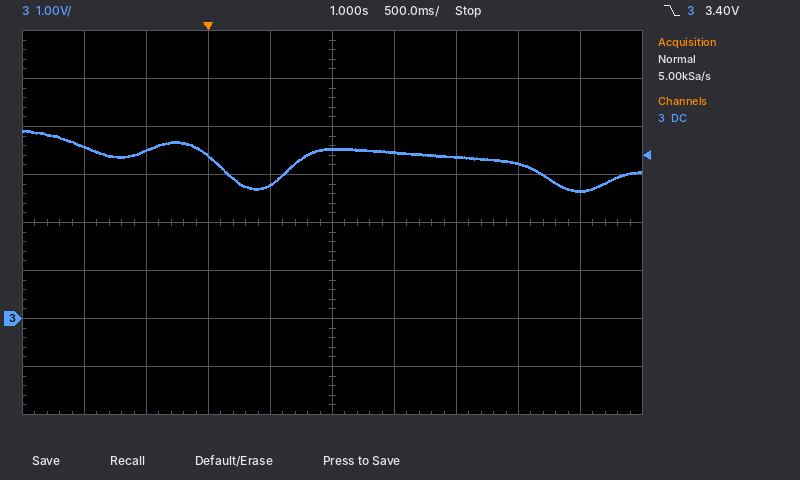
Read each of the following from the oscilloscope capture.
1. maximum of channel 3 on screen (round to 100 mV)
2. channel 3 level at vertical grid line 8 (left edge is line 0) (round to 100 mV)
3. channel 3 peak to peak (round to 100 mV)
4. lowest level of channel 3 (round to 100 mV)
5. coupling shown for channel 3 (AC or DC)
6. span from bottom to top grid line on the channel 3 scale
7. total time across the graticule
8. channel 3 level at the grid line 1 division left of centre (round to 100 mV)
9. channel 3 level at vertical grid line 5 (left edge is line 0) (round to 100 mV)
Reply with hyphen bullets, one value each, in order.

- 3.9 V
- 3.2 V
- 1.3 V
- 2.6 V
- DC
- 8 V
- 5 s
- 2.8 V
- 3.5 V
